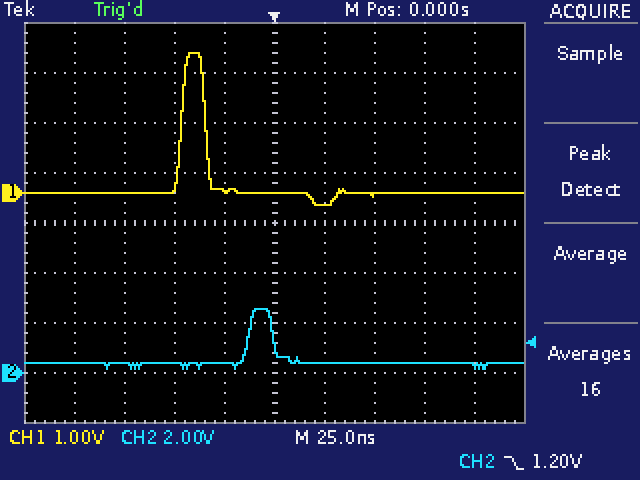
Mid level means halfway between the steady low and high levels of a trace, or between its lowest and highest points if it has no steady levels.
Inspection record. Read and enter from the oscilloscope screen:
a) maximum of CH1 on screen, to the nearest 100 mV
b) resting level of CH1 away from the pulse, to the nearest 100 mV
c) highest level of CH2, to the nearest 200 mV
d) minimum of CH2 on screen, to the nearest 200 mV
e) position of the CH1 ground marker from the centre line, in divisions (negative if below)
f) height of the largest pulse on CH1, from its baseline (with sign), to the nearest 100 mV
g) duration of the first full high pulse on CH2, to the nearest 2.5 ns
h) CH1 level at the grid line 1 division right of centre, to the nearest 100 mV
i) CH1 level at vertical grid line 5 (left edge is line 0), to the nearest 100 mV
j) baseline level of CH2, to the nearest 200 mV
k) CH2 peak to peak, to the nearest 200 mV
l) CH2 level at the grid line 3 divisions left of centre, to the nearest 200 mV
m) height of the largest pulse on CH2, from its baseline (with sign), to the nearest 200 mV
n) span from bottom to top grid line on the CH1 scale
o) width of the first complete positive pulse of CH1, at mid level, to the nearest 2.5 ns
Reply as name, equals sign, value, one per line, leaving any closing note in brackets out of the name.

maximum of CH1 on screen, to the nearest 100 mV = 2.8 V
resting level of CH1 away from the pulse, to the nearest 100 mV = 0.0 V
highest level of CH2, to the nearest 200 mV = 2.6 V
minimum of CH2 on screen, to the nearest 200 mV = 200 mV
position of the CH1 ground marker from the centre line, in divisions = +0.6 div
height of the largest pulse on CH1, from its baseline (with sign), to the nearest 100 mV = +2.8 V
duration of the first full high pulse on CH2, to the nearest 2.5 ns = 12.5 ns
CH1 level at the grid line 1 division right of centre, to the nearest 100 mV = -200 mV
CH1 level at vertical grid line 5 (left edge is line 0), to the nearest 100 mV = 0.0 V
baseline level of CH2, to the nearest 200 mV = 400 mV
CH2 peak to peak, to the nearest 200 mV = 2.4 V
CH2 level at the grid line 3 divisions left of centre, to the nearest 200 mV = 400 mV
height of the largest pulse on CH2, from its baseline (with sign), to the nearest 200 mV = +2.2 V
span from bottom to top grid line on the CH1 scale = 8 V
width of the first complete positive pulse of CH1, at mid level, to the nearest 2.5 ns = 12.5 ns
